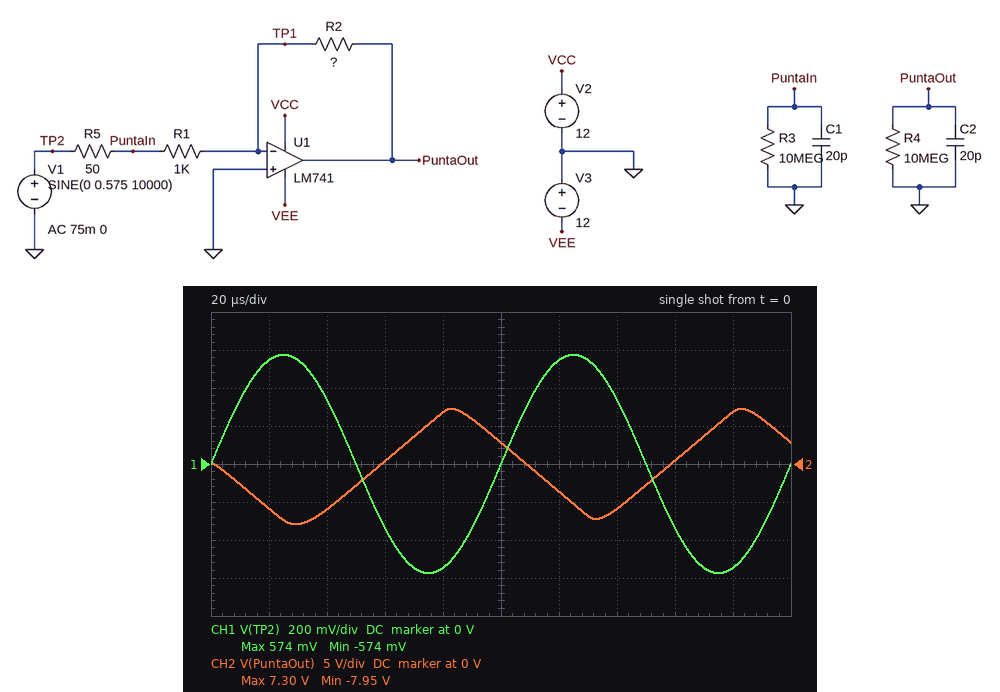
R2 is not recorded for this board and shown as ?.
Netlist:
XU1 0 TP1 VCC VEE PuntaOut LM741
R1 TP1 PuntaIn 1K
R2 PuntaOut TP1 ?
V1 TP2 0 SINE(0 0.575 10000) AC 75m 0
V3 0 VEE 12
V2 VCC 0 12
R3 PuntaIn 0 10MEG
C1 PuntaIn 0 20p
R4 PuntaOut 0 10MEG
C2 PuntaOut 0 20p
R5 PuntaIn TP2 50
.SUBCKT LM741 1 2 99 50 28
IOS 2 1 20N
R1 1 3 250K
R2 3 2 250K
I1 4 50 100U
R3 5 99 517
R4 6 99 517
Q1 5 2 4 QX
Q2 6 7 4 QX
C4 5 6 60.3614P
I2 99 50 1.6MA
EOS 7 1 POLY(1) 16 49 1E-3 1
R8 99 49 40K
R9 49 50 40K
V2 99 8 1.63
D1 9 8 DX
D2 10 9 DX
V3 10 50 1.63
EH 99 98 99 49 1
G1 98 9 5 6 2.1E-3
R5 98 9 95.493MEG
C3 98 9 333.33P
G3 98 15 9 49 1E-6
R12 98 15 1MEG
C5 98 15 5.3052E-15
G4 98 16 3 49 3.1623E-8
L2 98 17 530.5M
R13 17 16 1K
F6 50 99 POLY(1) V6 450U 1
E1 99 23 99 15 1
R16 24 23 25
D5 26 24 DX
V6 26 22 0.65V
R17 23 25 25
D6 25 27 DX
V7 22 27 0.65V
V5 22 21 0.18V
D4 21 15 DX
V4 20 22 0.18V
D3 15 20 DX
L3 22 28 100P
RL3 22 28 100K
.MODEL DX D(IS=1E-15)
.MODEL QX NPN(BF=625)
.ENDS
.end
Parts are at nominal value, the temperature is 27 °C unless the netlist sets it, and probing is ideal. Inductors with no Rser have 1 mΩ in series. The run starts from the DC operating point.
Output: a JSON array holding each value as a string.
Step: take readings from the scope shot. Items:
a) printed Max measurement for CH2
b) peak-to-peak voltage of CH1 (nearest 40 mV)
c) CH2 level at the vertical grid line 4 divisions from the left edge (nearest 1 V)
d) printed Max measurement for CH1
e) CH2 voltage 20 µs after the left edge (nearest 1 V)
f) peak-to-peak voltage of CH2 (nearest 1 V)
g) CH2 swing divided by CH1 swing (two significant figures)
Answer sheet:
["7.30 V", "1.16 V", "7 V", "574 mV", "-6 V", "15 V", "13"]
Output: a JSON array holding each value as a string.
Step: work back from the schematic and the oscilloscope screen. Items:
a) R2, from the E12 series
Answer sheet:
["15 kΩ"]
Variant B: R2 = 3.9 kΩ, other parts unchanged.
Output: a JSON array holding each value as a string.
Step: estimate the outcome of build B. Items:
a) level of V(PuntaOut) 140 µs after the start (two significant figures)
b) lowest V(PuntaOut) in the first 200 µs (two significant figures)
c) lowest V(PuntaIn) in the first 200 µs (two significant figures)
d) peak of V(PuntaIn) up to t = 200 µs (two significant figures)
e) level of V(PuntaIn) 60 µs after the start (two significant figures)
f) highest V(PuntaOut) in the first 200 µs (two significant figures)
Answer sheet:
["-1.3 V", "-2.1 V", "-550 mV", "550 mV", "-320 mV", "2.1 V"]
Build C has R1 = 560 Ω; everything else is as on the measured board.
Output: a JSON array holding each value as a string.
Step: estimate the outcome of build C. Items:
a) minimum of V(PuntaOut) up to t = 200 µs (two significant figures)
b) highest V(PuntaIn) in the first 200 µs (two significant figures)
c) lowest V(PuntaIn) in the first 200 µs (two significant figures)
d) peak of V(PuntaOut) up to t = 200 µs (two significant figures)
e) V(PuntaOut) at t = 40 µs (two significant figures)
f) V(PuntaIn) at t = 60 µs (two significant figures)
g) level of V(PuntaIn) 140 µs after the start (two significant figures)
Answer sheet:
["-11 V", "560 mV", "-570 mV", "7.5 V", "-10 V", "-350 mV", "310 mV"]
